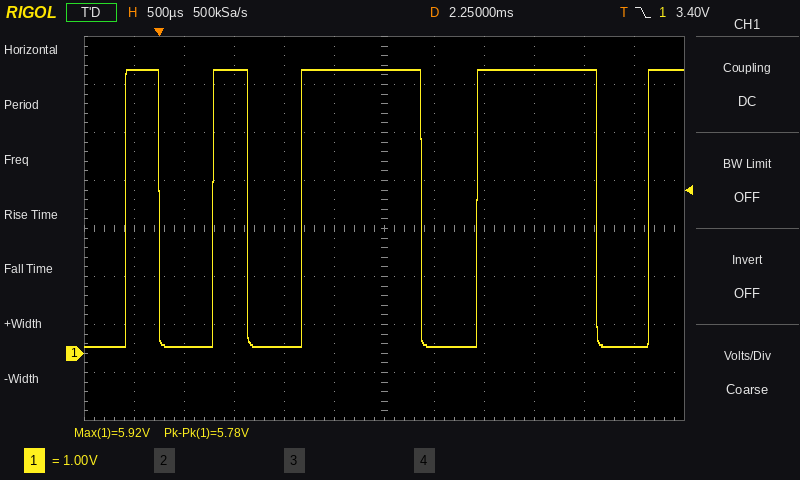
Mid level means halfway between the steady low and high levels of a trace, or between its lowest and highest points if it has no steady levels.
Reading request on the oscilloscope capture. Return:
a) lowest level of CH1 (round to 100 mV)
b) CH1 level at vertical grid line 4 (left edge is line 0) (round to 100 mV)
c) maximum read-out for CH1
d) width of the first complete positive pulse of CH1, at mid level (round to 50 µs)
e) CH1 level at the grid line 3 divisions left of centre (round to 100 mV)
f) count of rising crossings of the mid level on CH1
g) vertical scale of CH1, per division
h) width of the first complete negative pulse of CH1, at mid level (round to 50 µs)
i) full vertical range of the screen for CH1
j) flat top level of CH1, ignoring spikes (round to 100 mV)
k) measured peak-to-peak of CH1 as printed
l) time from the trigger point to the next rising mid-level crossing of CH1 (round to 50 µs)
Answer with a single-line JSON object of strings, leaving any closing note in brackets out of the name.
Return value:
{"lowest level of CH1": "100 mV", "CH1 level at vertical grid line 4 (left edge is line 0)": "100 mV", "maximum read-out for CH1": "5.92 V", "width of the first complete positive pulse of CH1, at mid level": "350 µs", "CH1 level at the grid line 3 divisions left of centre": "5.9 V", "count of rising crossings of the mid level on CH1": "5", "vertical scale of CH1, per division": "1 V", "width of the first complete negative pulse of CH1, at mid level": "550 µs", "full vertical range of the screen for CH1": "8 V", "flat top level of CH1, ignoring spikes": "5.9 V", "measured peak-to-peak of CH1 as printed": "5.78 V", "time from the trigger point to the next rising mid-level crossing of CH1": "550 µs"}
